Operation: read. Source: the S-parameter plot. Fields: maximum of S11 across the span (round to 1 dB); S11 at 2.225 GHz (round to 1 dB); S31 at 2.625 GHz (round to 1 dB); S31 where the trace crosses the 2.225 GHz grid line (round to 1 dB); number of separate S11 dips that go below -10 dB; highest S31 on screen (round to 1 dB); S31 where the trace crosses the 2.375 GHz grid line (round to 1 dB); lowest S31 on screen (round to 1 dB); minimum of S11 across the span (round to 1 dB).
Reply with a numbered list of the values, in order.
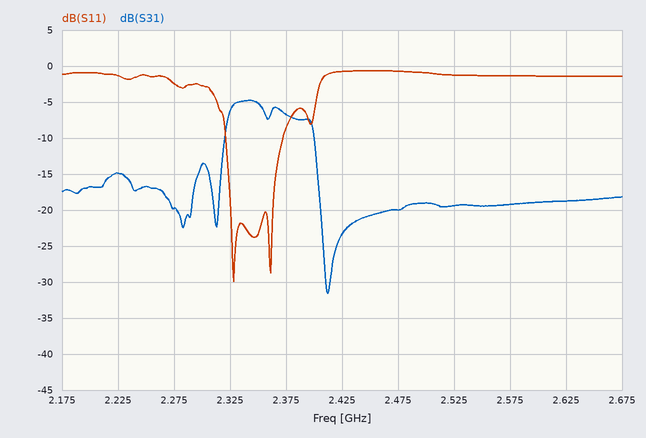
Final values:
1. -1 dB
2. -1 dB
3. -19 dB
4. -15 dB
5. 2
6. -5 dB
7. -7 dB
8. -32 dB
9. -30 dB
